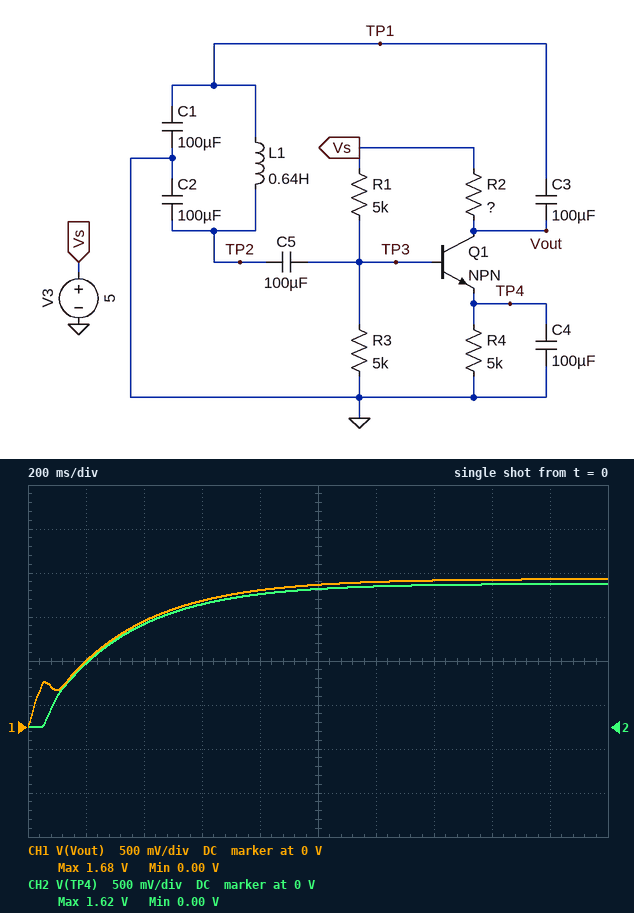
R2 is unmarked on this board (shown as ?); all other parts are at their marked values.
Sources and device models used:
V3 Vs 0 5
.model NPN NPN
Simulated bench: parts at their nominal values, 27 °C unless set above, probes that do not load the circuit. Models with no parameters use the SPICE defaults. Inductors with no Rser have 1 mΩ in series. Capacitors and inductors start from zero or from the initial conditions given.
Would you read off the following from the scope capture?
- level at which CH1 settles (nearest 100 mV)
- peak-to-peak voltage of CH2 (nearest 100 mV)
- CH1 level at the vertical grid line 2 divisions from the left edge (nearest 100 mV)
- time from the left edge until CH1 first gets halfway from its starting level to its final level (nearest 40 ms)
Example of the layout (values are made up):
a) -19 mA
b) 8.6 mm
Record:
a) 1.7 V
b) 1.6 V
c) 1.2 V
d) 240 ms
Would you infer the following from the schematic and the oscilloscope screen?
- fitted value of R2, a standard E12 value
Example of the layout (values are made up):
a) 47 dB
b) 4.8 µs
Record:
a) 12 kΩ
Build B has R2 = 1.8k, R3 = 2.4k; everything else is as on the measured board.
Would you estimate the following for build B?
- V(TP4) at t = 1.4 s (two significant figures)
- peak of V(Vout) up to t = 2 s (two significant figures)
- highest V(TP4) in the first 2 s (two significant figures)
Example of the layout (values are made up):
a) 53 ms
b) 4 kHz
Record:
a) 1.2 V
b) 4.9 V
c) 1.3 V
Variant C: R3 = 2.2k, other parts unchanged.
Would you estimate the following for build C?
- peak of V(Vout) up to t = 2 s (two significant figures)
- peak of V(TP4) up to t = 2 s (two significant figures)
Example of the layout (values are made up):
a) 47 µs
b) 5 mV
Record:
a) 2.5 V
b) 1.3 V
